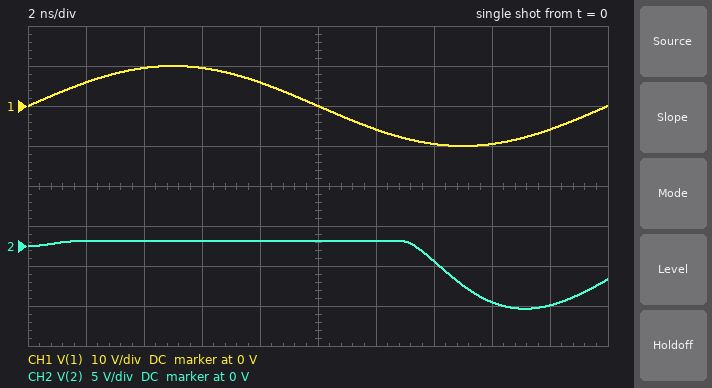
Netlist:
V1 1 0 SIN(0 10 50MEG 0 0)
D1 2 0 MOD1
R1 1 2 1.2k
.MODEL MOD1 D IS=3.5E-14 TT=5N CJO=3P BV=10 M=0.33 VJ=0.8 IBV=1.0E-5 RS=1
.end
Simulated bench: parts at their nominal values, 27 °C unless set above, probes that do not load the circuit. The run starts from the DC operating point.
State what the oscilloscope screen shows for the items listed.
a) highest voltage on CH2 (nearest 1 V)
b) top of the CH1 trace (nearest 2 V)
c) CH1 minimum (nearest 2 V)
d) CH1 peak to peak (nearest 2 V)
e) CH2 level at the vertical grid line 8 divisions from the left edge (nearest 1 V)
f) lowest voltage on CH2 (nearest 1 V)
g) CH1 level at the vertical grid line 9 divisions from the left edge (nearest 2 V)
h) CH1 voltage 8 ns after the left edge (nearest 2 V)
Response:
1 V
10 V
-10 V
20 V
-7 V
-8 V
-6 V
6 V
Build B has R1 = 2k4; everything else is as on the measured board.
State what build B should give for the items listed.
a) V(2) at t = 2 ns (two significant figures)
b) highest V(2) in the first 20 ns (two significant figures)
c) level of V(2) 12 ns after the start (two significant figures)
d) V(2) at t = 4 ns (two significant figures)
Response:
560 mV
650 mV
610 mV
630 mV
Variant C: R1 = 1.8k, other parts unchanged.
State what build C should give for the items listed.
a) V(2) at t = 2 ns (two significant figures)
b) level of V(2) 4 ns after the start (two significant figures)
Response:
580 mV
640 mV
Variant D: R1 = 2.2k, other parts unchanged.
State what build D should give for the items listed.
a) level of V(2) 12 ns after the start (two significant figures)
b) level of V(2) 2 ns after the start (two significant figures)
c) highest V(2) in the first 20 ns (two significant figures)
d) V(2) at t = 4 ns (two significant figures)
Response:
610 mV
570 mV
650 mV
630 mV
